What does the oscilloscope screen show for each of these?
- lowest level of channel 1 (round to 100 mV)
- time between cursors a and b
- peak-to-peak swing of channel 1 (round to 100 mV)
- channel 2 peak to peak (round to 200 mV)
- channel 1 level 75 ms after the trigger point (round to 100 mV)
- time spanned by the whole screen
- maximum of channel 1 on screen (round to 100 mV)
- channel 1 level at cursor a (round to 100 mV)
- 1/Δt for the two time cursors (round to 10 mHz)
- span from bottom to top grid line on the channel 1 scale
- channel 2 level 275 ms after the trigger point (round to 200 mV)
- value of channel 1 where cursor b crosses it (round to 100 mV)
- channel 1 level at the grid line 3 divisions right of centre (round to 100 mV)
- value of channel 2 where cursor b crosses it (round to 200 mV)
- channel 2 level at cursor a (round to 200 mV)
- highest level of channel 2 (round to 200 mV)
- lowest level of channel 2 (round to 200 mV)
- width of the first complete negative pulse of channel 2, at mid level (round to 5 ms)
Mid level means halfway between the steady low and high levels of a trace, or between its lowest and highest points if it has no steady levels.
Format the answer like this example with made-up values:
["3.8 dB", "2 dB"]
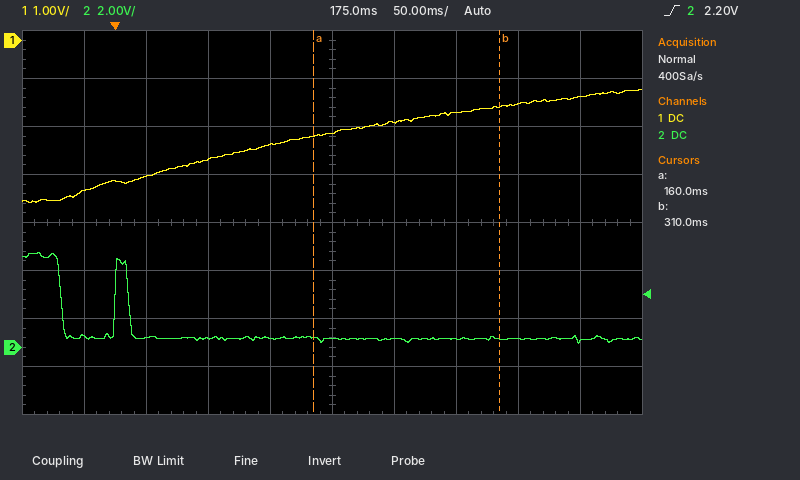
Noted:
["-3.4 V", "150 ms", "2.4 V", "3.8 V", "-2.5 V", "500 ms", "-1.0 V", "-2.0 V", "6.67 Hz", "8 V", "400 mV", "-1.4 V", "-1.3 V", "400 mV", "400 mV", "4.0 V", "200 mV", "45 ms"]
